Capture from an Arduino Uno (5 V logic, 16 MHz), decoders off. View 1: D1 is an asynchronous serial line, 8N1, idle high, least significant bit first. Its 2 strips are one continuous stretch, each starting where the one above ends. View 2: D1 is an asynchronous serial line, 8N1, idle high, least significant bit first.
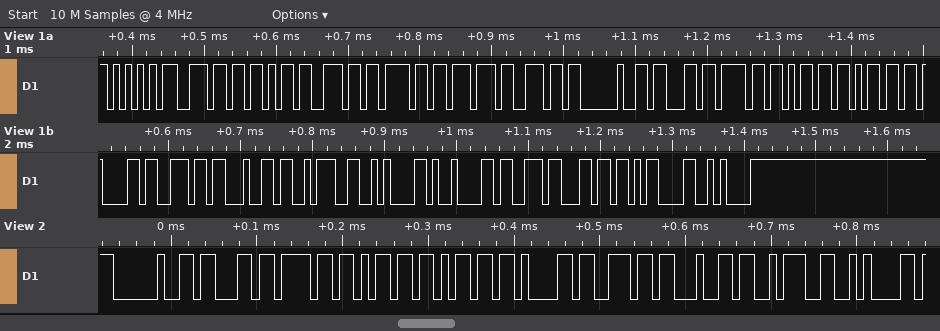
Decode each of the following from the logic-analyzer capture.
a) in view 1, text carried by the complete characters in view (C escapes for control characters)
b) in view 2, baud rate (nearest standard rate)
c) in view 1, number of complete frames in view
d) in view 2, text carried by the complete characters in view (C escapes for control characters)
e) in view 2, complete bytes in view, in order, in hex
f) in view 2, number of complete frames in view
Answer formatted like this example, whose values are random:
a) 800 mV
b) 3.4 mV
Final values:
a) "Unknown command:\n\tsl\r\n"
b) 115200 baud
c) 22
d) " command:\n"
e) 20 63 6F 6D 6D 61 6E 64 3A 0A
f) 10
